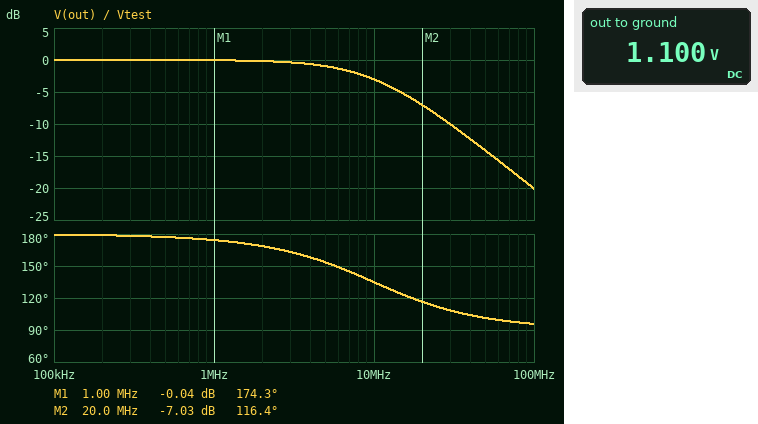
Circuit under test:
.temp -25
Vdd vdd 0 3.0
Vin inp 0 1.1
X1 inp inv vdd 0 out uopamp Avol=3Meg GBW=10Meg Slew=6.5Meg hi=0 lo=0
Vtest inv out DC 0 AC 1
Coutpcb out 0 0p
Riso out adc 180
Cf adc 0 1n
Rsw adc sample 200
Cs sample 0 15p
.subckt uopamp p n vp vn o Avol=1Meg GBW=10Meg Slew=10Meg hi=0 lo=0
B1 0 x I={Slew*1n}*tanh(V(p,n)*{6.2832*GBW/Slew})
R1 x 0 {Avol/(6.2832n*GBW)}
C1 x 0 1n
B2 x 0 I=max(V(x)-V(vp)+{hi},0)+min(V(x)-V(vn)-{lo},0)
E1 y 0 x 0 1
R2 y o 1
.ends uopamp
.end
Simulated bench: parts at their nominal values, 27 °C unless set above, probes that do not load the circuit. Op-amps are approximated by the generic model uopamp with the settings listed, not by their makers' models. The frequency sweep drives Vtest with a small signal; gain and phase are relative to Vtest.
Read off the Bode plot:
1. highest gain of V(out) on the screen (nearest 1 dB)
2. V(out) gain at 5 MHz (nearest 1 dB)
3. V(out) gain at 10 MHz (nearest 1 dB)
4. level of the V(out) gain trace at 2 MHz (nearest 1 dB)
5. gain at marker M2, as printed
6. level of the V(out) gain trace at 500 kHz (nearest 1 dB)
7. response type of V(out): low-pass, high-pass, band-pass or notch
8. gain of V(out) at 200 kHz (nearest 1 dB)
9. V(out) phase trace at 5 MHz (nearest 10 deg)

0 dB
-1 dB
-3 dB
0 dB
-7.03 dB
0 dB
low-pass
0 dB
150 deg
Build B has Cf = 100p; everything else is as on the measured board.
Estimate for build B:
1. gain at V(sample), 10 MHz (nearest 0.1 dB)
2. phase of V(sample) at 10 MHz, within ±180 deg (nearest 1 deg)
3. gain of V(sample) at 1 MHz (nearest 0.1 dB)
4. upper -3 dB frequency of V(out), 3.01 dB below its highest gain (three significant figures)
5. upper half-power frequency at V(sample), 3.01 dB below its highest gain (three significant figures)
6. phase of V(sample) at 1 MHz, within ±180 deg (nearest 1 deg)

-7.5 dB
73 deg
-0.1 dB
9.99 MHz
5.47 MHz
166 deg
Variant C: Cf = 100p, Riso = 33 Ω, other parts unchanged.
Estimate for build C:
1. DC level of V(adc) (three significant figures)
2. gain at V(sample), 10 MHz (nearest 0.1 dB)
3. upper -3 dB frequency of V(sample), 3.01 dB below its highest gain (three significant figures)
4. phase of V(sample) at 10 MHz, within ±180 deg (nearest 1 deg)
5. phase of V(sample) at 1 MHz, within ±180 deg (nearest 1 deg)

1.10 V
-3.4 dB
9.19 MHz
111 deg
172 deg
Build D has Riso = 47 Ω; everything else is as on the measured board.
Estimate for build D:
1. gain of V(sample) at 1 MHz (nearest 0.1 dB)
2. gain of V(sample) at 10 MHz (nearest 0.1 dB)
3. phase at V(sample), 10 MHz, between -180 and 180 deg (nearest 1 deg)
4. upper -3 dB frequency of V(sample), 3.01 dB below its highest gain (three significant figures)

-0.4 dB
-13.2 dB
52 deg
3.04 MHz
